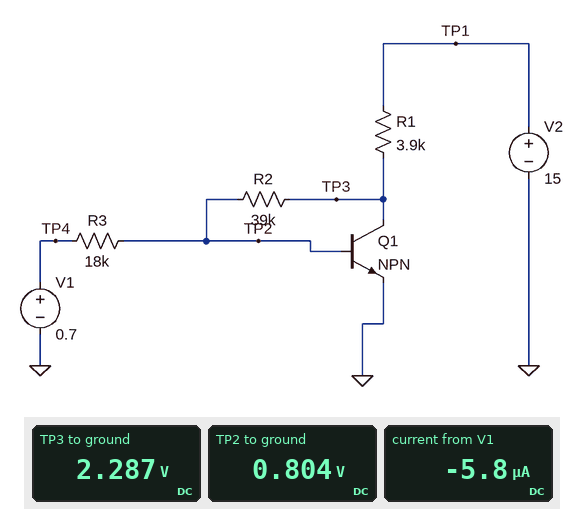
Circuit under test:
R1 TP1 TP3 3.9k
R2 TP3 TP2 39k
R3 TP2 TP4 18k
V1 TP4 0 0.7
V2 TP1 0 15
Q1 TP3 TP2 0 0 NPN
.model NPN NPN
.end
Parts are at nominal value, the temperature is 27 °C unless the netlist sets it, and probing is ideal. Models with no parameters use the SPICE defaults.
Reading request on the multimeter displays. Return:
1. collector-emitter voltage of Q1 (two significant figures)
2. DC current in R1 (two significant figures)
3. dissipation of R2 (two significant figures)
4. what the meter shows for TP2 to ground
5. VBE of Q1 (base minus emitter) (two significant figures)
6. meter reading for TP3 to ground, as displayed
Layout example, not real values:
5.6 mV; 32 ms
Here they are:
2.3 V; 3.3 mA; 56 µW; 0.804 V; 800 mV; 2.287 V
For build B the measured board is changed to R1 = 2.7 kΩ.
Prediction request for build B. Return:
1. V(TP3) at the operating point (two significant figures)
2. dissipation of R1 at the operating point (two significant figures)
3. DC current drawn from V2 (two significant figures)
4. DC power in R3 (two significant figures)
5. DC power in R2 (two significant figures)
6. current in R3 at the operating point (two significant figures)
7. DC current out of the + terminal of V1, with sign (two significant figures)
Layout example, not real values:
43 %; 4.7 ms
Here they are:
2.8 V; 55 mW; 4.5 mA; 710 nW; 100 µW; 6.3 µA; -6.3 µA
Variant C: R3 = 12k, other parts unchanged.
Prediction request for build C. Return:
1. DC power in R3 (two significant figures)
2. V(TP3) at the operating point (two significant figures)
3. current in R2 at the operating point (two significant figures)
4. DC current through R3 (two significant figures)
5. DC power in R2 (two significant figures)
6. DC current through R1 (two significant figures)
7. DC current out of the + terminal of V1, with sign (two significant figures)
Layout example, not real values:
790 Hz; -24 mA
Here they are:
910 nW; 2.4 V; 41 µA; 8.7 µA; 64 µW; 3.2 mA; -8.7 µA
